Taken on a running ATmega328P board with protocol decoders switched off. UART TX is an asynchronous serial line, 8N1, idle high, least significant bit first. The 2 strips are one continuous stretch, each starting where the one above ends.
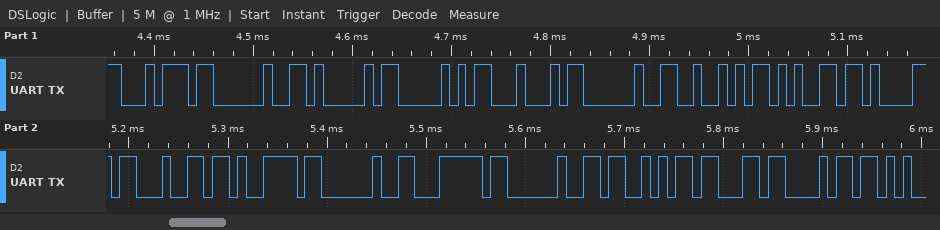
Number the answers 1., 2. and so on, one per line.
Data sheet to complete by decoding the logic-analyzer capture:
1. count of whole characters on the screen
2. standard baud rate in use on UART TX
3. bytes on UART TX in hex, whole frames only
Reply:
1. 17
2. 115200 baud
3. 74 20 41 50 44 20 52 65 61 64 79 20 7C 20 53 63 68
